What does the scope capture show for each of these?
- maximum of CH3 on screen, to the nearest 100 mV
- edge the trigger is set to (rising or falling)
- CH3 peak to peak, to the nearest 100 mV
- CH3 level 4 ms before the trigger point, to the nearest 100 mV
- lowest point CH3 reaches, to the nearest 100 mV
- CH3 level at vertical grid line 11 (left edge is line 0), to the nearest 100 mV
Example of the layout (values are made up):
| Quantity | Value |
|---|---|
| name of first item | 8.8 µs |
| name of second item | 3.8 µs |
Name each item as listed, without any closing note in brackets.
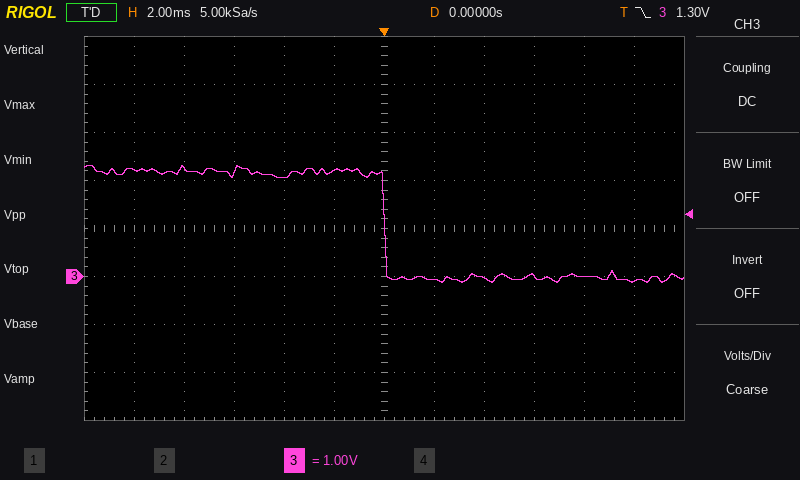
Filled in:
| Quantity | Value |
|---|---|
| maximum of CH3 on screen, to the nearest 100 mV | 2.3 V |
| edge the trigger is set to | falling |
| CH3 peak to peak, to the nearest 100 mV | 2.4 V |
| CH3 level 4 ms before the trigger point, to the nearest 100 mV | 2.1 V |
| lowest point CH3 reaches, to the nearest 100 mV | -100 mV |
| CH3 level at vertical grid line 11 (left edge is line 0), to the nearest 100 mV | -100 mV |
